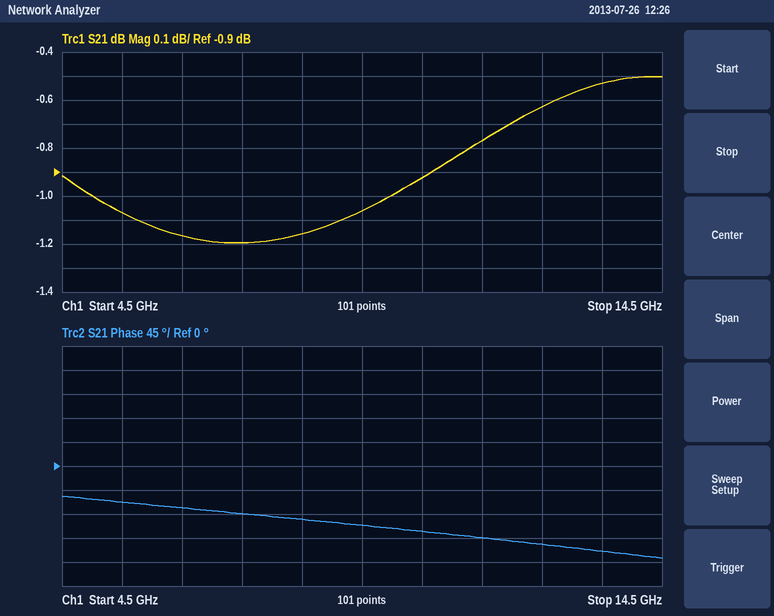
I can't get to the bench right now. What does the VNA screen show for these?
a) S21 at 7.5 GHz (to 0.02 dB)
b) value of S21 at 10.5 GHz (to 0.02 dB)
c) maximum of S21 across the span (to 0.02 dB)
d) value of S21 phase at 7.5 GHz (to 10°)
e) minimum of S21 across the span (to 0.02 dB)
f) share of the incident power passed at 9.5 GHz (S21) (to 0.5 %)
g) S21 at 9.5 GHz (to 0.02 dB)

-1.20 dB
-0.92 dB
-0.50 dB
-90°
-1.20 dB
78.5 %
-1.06 dB
